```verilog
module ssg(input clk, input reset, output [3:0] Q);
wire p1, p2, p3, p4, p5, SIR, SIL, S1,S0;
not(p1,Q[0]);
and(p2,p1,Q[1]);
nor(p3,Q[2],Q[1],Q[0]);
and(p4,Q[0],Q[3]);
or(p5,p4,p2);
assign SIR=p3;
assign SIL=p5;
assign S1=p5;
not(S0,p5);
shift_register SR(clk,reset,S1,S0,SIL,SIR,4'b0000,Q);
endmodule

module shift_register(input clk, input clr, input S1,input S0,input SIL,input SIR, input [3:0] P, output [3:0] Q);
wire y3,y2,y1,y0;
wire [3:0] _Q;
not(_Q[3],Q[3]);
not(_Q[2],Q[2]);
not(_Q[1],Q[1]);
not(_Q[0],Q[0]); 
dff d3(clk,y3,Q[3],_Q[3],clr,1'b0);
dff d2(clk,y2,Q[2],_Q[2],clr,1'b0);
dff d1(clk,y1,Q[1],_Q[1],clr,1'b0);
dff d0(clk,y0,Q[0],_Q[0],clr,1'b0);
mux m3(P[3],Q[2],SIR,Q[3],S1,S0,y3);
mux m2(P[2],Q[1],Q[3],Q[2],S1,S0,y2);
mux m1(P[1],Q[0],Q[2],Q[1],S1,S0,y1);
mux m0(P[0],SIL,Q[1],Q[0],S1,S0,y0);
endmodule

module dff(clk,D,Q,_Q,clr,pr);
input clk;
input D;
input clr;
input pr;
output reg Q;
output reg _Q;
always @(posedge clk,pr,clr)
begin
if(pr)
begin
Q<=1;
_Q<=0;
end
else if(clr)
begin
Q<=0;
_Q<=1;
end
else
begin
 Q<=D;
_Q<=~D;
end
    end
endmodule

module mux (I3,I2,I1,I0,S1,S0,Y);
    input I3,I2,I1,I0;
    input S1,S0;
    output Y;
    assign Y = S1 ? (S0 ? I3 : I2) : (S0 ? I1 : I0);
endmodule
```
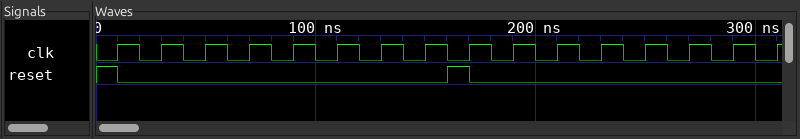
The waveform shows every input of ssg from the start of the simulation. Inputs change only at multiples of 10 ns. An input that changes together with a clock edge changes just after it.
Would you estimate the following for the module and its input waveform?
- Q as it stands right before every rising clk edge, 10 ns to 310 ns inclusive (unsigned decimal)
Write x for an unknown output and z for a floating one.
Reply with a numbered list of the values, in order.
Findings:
1. 0, 8, 12, 6, 13, 11, 7, 3, 0, 8, 12, 6, 13, 11, 7, 3
